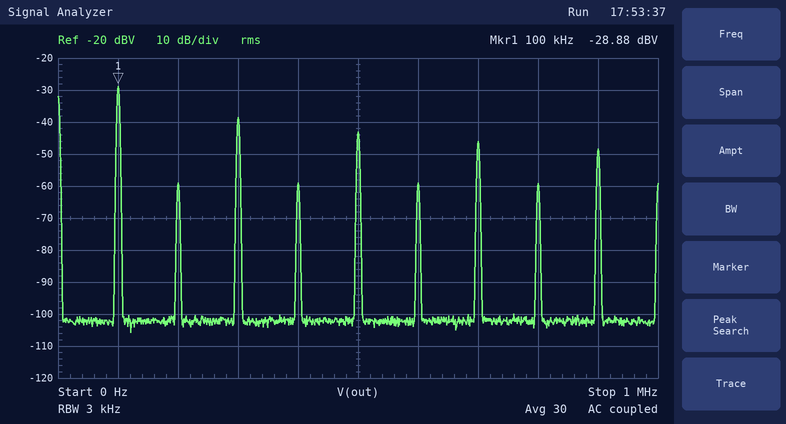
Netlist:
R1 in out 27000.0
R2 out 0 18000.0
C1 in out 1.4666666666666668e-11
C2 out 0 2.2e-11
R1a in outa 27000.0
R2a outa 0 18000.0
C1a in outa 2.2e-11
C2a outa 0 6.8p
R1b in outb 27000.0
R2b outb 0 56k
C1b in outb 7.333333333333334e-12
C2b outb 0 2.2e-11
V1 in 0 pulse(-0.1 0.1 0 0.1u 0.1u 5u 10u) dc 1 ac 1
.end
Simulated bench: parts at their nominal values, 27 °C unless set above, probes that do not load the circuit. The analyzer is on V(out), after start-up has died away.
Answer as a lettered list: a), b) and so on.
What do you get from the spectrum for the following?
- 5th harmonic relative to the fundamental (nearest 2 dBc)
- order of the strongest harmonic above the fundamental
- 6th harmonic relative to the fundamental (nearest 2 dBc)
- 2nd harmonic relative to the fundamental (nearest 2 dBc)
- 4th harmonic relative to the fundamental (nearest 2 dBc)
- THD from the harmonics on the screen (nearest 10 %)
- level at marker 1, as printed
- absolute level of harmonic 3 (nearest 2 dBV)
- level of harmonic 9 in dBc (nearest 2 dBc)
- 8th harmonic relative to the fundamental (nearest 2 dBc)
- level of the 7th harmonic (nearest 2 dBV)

a) -14 dBc
b) 3
c) -30 dBc
d) -30 dBc
e) -30 dBc
f) 40 %
g) -28.88 dBV
h) -38 dBV
i) -20 dBc
j) -30 dBc
k) -46 dBV
